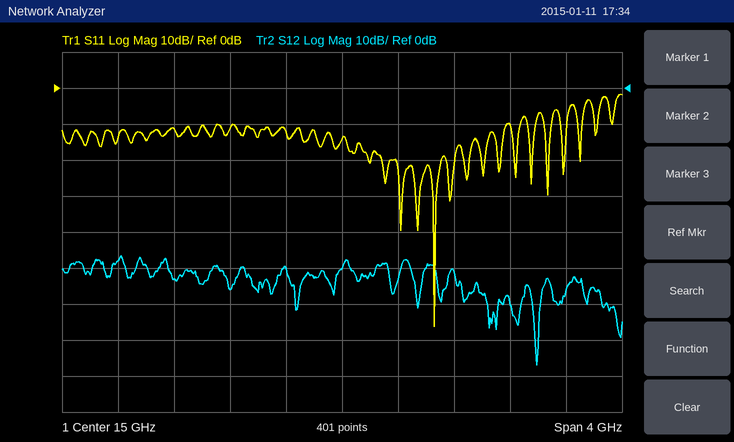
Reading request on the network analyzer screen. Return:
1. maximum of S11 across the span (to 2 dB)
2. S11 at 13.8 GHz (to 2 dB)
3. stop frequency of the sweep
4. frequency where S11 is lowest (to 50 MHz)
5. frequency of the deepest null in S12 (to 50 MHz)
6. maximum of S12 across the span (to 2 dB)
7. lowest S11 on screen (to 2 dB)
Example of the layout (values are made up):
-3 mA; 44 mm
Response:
-2 dB; -12 dB; 17 GHz; 15.65 GHz; 16.40 GHz; -46 dB; -66 dB
